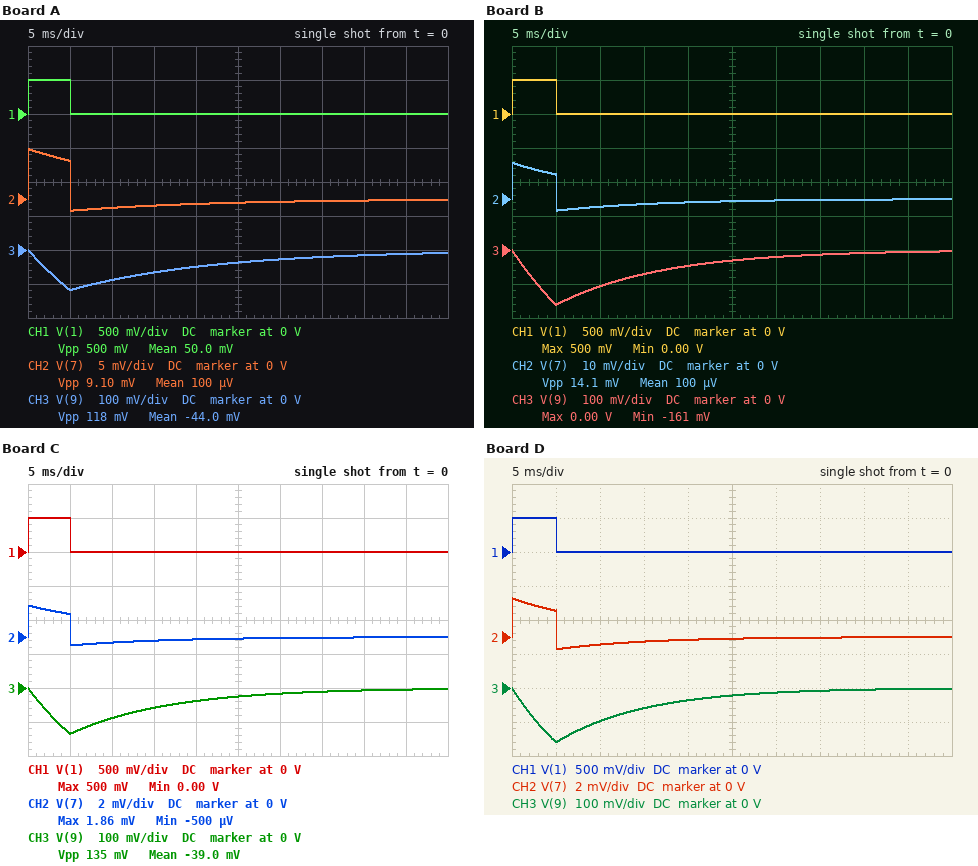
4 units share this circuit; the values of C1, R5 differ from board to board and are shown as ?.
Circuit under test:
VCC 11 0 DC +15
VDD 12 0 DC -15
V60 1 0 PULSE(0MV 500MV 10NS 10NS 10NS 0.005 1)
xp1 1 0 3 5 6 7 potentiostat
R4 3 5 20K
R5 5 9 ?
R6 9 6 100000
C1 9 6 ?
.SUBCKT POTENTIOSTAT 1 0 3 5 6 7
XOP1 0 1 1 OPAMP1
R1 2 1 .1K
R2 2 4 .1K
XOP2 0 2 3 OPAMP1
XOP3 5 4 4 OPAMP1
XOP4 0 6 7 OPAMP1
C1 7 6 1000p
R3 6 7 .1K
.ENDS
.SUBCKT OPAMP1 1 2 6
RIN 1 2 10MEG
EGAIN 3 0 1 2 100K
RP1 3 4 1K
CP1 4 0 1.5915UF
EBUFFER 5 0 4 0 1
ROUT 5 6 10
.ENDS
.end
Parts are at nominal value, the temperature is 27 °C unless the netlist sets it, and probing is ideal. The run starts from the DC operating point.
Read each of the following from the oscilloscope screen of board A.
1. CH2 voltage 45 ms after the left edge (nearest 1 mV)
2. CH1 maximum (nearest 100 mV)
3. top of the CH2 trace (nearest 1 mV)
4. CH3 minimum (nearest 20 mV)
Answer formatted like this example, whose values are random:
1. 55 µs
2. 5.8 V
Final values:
1. 0 V
2. 500 mV
3. 7 mV
4. -120 mV
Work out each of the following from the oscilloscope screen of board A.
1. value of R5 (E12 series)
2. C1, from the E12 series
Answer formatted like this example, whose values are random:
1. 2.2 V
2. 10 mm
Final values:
1. 6.8 kΩ
2. 2.7 µF
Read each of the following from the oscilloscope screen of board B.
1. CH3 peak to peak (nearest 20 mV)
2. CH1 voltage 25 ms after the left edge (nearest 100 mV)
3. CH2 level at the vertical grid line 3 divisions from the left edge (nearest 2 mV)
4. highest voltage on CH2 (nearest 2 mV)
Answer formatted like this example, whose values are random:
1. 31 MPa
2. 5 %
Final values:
1. 160 mV
2. 0 V
3. -2 mV
4. 10 mV
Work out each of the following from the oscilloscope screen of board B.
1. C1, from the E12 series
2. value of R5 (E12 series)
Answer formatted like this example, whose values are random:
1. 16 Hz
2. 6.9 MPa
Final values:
1. 2.7 µF
2. 4.7 kΩ
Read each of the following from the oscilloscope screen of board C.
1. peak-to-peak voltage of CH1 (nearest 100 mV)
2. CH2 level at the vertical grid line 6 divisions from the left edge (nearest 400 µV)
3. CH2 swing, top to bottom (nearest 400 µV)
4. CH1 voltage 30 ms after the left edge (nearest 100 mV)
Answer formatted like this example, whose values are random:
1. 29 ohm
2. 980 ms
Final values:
1. 500 mV
2. 0 V
3. 2.4 mV
4. 0 V
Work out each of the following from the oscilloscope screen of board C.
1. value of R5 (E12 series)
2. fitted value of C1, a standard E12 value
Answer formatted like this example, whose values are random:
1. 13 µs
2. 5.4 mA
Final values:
1. 27 kΩ
2. 560 nF
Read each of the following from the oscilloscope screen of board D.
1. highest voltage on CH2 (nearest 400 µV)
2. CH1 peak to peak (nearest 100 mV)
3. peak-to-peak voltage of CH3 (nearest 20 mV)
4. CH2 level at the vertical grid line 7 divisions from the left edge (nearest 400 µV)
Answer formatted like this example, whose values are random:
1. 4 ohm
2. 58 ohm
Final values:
1. 2.4 mV
2. 500 mV
3. 160 mV
4. 0 V
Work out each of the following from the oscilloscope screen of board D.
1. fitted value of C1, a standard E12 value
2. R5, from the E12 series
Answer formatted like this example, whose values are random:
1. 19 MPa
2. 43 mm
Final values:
1. 560 nF
2. 22 kΩ
